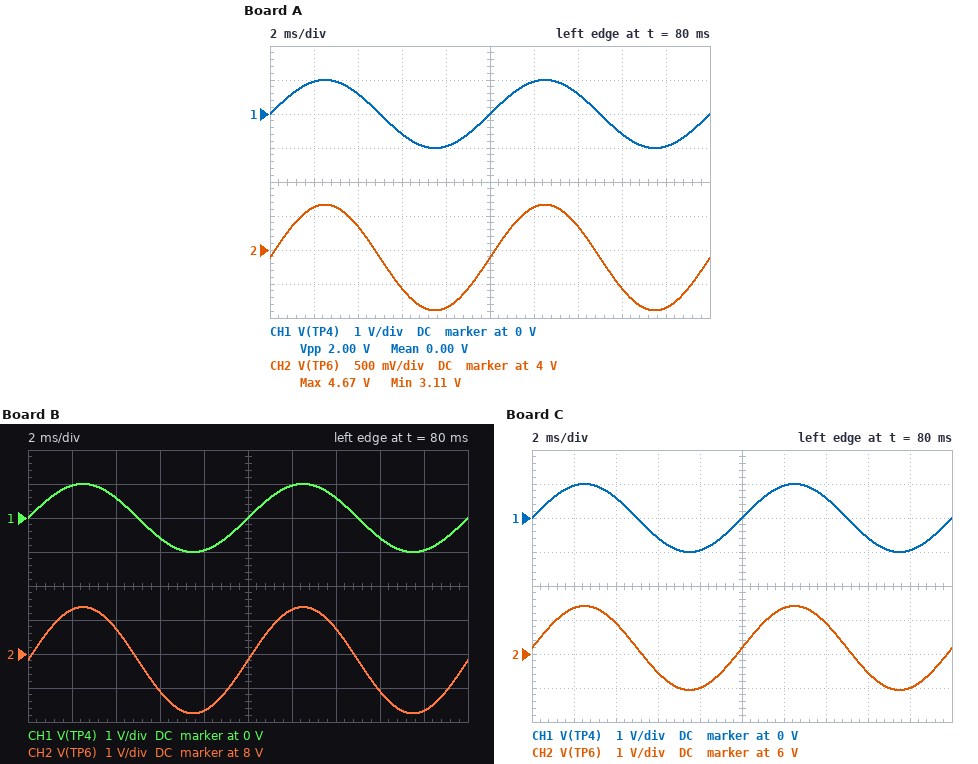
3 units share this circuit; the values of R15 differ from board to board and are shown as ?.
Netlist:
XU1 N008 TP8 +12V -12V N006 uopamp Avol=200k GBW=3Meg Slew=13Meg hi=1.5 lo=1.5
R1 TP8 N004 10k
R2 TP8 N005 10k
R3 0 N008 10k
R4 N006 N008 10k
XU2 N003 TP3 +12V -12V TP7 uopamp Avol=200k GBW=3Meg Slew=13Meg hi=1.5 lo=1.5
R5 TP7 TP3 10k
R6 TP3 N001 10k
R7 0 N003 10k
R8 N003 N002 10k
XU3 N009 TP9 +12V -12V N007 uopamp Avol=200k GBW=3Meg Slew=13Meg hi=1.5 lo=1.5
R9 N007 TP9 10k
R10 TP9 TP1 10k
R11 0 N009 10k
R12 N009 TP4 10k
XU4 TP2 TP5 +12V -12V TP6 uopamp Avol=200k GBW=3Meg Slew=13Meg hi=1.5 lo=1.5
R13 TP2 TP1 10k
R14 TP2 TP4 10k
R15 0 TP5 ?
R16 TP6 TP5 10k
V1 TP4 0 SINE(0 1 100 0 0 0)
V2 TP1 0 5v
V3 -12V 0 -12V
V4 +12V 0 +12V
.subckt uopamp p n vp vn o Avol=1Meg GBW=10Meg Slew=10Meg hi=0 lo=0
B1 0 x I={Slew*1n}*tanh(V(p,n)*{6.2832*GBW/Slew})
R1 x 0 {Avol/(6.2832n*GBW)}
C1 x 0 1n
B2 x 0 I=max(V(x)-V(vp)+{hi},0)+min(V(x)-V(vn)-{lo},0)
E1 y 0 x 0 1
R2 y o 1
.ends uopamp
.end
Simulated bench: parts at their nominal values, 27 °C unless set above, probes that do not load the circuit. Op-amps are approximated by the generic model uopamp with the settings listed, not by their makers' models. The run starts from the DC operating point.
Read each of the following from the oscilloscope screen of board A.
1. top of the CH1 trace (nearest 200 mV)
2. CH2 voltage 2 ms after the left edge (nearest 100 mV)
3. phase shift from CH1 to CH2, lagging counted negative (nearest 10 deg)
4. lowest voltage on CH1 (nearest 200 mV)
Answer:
1.0 V
4.6 V
0 deg
-1.0 V
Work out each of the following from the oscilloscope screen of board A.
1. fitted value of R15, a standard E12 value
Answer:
18 kΩ
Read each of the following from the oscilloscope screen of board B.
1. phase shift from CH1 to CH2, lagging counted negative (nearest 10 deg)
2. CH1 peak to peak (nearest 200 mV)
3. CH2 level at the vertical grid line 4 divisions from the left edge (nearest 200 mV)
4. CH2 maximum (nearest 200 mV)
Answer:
0 deg
2.0 V
6.4 V
9.4 V
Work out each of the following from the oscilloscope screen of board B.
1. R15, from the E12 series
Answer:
4.7 kΩ
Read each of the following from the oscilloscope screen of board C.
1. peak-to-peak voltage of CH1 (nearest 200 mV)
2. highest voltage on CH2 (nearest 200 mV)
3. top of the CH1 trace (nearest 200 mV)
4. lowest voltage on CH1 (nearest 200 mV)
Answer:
2.0 V
7.4 V
1.0 V
-1.0 V
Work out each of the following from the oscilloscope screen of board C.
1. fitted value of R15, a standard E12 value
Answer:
6.8 kΩ
